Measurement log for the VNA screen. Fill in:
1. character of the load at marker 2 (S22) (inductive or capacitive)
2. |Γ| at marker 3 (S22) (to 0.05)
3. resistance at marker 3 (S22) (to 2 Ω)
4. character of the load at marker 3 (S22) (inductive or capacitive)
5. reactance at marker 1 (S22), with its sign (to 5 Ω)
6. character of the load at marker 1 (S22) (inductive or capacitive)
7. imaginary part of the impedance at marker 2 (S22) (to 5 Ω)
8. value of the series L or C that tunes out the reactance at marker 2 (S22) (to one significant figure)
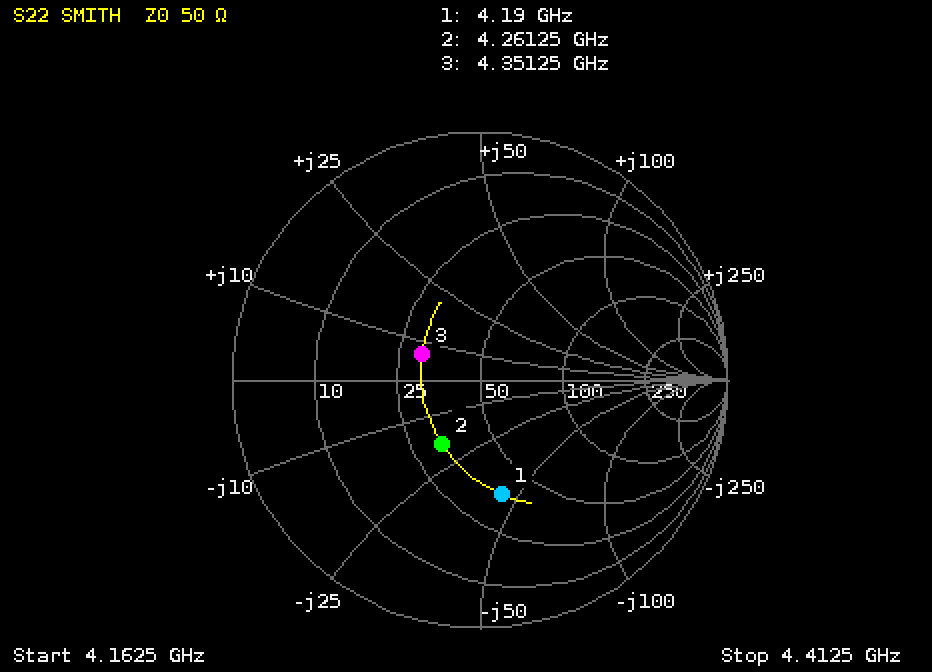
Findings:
capacitive
0.25
30 Ω
inductive
-45 Ω
capacitive
-20 Ω
700 pH
